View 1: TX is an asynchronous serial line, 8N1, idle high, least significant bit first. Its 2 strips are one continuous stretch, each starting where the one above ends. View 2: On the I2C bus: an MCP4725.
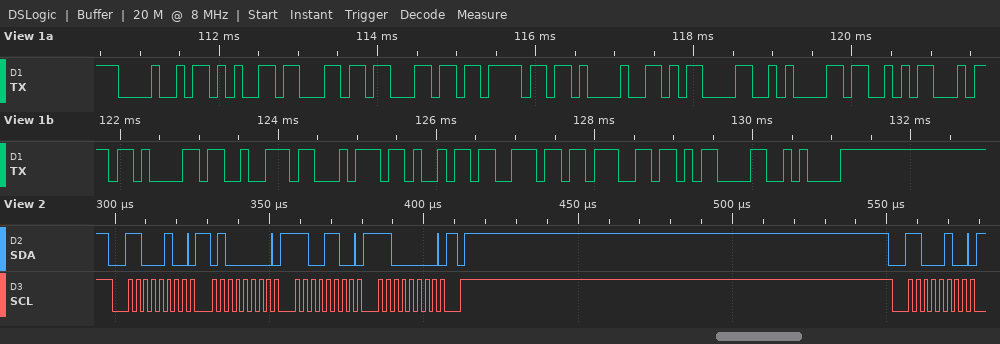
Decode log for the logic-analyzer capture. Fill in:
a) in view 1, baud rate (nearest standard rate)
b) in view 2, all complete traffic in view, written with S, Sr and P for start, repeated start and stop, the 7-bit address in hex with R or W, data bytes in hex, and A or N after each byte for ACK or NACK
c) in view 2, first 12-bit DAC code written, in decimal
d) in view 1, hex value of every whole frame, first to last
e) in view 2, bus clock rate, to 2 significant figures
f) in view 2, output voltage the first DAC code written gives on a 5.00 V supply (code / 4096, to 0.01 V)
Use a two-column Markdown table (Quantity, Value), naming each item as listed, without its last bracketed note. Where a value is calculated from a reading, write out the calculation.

| Quantity | Value |
|---|---|
| in view 1, baud rate | 9600 baud |
| in view 2, all complete traffic in view, written with S, Sr and P for start, repeated start and stop, the 7-bit address in hex with R or W, data bytes in hex, and A or N after each byte for ACK or NACK | S 62W A 40 A CC A C0 A P S 62W A |
| in view 2, first 12-bit DAC code written, in decimal | 3276 |
| in view 1, hex value of every whole frame, first to last | 48 65 6C 6C 6F 21 0D 0A 53 74 61 72 74 69 6E 67 0D 0A |
| in view 2, bus clock rate, to 2 significant figures | 400 kHz |
| in view 2, output voltage the first DAC code written gives on a 5.00 V supply | 3276 / 4096 x 5.00 V = 4.00 V |
